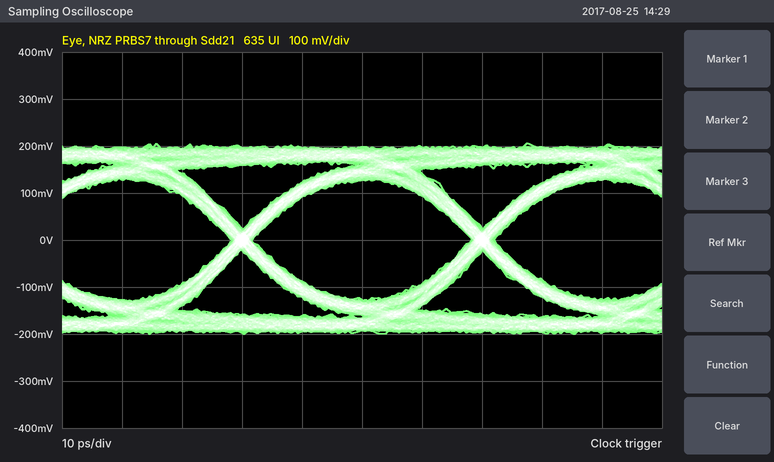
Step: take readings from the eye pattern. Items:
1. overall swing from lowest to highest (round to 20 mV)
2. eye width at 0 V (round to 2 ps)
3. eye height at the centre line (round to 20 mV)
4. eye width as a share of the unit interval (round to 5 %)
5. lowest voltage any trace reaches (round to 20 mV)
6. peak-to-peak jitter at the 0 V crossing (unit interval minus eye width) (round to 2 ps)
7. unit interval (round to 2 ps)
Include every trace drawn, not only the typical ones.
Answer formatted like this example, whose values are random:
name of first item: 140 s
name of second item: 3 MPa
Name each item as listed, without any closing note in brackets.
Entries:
overall swing from lowest to highest: 400 mV
eye width at 0 V: 36 ps
eye height at the centre line: 260 mV
eye width as a share of the unit interval: 90 %
lowest voltage any trace reaches: -200 mV
peak-to-peak jitter at the 0 V crossing (unit interval minus eye width): 4 ps
unit interval: 40 ps
